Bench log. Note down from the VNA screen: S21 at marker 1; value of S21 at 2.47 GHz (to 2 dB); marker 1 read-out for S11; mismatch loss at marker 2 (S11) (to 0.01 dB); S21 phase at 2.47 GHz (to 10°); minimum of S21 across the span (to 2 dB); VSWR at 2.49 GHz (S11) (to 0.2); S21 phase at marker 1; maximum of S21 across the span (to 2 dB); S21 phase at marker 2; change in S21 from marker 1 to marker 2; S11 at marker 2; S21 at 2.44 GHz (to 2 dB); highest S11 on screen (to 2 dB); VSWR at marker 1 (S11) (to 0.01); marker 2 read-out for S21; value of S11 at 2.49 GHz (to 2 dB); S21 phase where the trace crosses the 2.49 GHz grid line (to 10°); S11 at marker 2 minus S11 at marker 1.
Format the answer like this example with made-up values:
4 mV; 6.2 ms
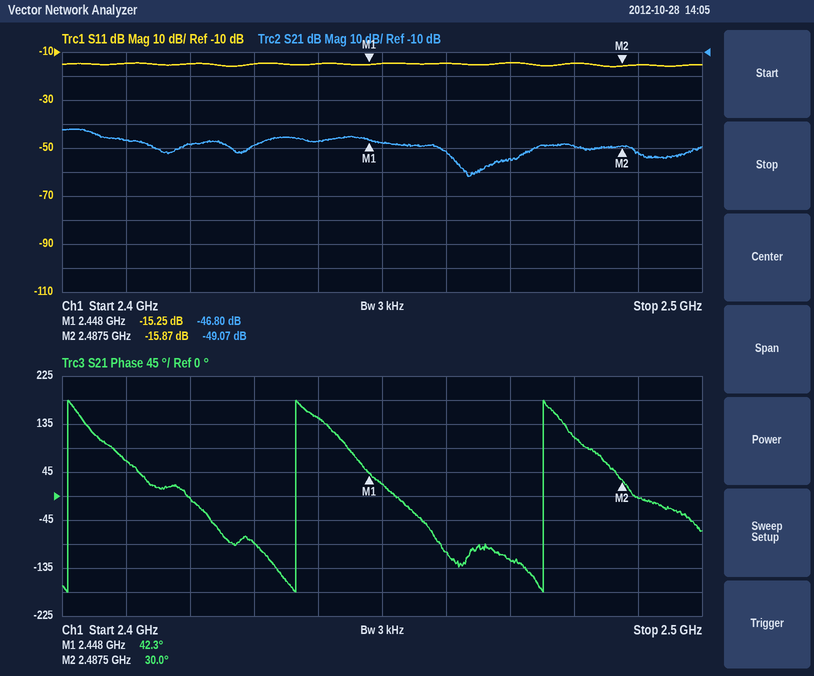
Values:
-46.80 dB; -54 dB; -15.25 dB; 0.11 dB; -120°; -62 dB; 1.4; 42.3°; -42 dB; 30.0°; -2.27 dB; -15.87 dB; -48 dB; -14 dB; 1.42; -49.07 dB; -16 dB; 0°; -0.62 dB
